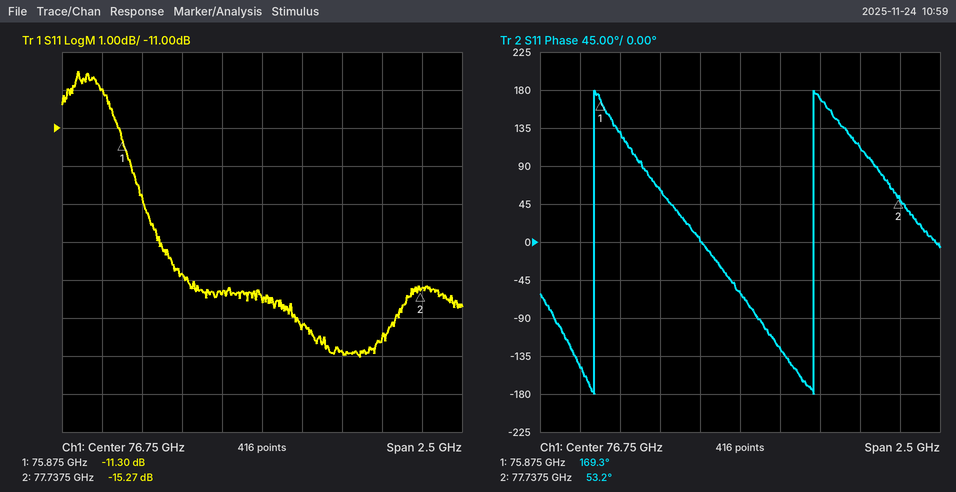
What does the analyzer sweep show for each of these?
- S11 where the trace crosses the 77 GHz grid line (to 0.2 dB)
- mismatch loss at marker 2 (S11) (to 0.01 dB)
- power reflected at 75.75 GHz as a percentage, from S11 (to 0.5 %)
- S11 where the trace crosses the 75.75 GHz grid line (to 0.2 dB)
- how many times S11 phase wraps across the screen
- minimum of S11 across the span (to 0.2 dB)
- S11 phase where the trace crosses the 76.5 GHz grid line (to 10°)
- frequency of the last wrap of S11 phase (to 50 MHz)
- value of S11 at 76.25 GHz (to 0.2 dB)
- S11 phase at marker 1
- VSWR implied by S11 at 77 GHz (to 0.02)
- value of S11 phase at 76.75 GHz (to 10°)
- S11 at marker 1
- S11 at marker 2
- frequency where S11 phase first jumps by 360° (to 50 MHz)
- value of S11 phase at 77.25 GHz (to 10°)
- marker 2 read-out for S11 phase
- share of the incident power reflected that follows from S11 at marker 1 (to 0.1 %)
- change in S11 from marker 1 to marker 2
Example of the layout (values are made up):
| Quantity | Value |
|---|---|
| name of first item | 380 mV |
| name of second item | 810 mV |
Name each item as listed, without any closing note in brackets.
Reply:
| Quantity | Value |
|---|---|
| S11 where the trace crosses the 77 GHz grid line | -16.2 dB |
| mismatch loss at marker 2 (S11) | 0.13 dB |
| power reflected at 75.75 GHz as a percentage, from S11 | 10.0 % |
| S11 where the trace crosses the 75.75 GHz grid line | -10.0 dB |
| how many times S11 phase wraps across the screen | 2 |
| minimum of S11 across the span | -17.0 dB |
| S11 phase where the trace crosses the 76.5 GHz grid line | 0° |
| frequency of the last wrap of S11 phase | 77.20 GHz |
| value of S11 at 76.25 GHz | -14.8 dB |
| S11 phase at marker 1 | 169.3° |
| VSWR implied by S11 at 77 GHz | 1.36 |
| value of S11 phase at 76.75 GHz | -60° |
| S11 at marker 1 | -11.30 dB |
| S11 at marker 2 | -15.27 dB |
| frequency where S11 phase first jumps by 360° | 75.85 GHz |
| value of S11 phase at 77.25 GHz | 170° |
| marker 2 read-out for S11 phase | 53.2° |
| share of the incident power reflected that follows from S11 at marker 1 | 7.4 % |
| change in S11 from marker 1 to marker 2 | -3.97 dB |
